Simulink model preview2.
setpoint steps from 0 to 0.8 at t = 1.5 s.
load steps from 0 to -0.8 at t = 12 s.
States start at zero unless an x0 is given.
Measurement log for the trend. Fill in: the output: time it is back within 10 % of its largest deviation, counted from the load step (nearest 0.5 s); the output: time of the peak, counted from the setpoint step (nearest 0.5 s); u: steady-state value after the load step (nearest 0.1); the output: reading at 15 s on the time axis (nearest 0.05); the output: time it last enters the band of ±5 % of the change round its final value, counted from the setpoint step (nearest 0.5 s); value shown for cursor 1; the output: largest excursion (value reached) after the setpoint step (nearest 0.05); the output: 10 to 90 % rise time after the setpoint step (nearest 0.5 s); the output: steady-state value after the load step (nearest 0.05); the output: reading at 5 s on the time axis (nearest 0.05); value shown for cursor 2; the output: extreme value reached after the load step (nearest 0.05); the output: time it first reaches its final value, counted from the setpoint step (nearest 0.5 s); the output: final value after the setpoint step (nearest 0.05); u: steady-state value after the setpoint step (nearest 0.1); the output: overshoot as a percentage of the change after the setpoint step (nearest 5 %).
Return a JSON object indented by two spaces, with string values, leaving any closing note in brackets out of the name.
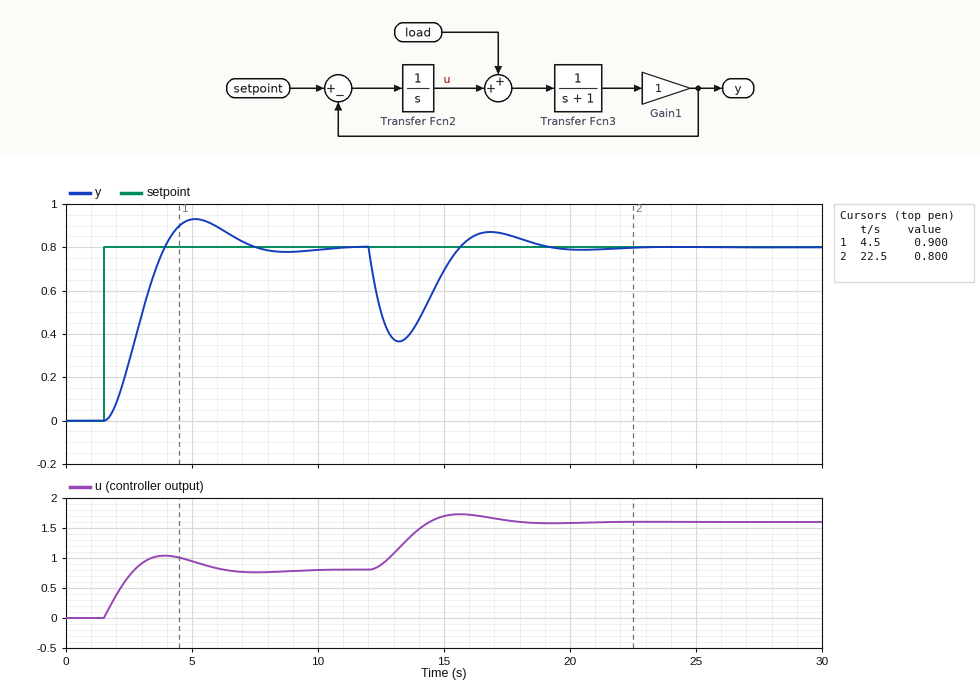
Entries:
{
  "the output: time it is back within 10 % of its largest deviation, counted from the load step": "6.0 s",
  "the output: time of the peak, counted from the setpoint step": "3.5 s",
  "u: steady-state value after the load step": "1.6",
  "the output: reading at 15 s on the time axis": "0.70",
  "the output: time it last enters the band of ±5 % of the change round its final value, counted from the setpoint step": "5.5 s",
  "value shown for cursor 1": "0.900",
  "the output: largest excursion (value reached) after the setpoint step": "0.95",
  "the output: 10 to 90 % rise time after the setpoint step": "1.5 s",
  "the output: steady-state value after the load step": "0.80",
  "the output: reading at 5 s on the time axis": "0.95",
  "value shown for cursor 2": "0.800",
  "the output: extreme value reached after the load step": "0.35",
  "the output: time it first reaches its final value, counted from the setpoint step": "2.5 s",
  "the output: final value after the setpoint step": "0.80",
  "u: steady-state value after the setpoint step": "0.8",
  "the output: overshoot as a percentage of the change after the setpoint step": "15 %"
}
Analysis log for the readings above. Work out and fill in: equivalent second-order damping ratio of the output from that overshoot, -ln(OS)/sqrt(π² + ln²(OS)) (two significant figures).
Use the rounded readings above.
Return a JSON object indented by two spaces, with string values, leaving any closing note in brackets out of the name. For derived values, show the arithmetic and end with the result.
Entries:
{
  "equivalent second-order damping ratio of the output from that overshoot, -ln(OS)/sqrt(π² + ln²(OS))": "ln(0.15) = -1.897; 1.897 / sqrt(9.870 + 3.599) = 0.52"
}
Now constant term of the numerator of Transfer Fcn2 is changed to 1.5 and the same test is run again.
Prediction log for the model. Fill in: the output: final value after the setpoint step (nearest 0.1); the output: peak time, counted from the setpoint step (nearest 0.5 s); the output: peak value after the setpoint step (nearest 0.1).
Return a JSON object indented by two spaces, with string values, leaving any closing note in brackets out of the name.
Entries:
{
  "the output: final value after the setpoint step": "0.8",
  "the output: peak time, counted from the setpoint step": "3.0 s",
  "the output: peak value after the setpoint step": "1.0"
}
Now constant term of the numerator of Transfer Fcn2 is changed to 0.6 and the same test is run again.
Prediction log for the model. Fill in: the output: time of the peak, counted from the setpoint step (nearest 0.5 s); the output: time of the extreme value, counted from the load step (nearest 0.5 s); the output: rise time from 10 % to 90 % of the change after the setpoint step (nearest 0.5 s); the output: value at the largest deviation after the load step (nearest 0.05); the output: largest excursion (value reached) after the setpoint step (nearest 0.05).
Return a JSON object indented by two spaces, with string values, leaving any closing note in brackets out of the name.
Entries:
{
  "the output: time of the peak, counted from the setpoint step": "5.5 s",
  "the output: time of the extreme value, counted from the load step": "1.5 s",
  "the output: rise time from 10 % to 90 % of the change after the setpoint step": "2.5 s",
  "the output: value at the largest deviation after the load step": "0.30",
  "the output: largest excursion (value reached) after the setpoint step": "0.85"
}
